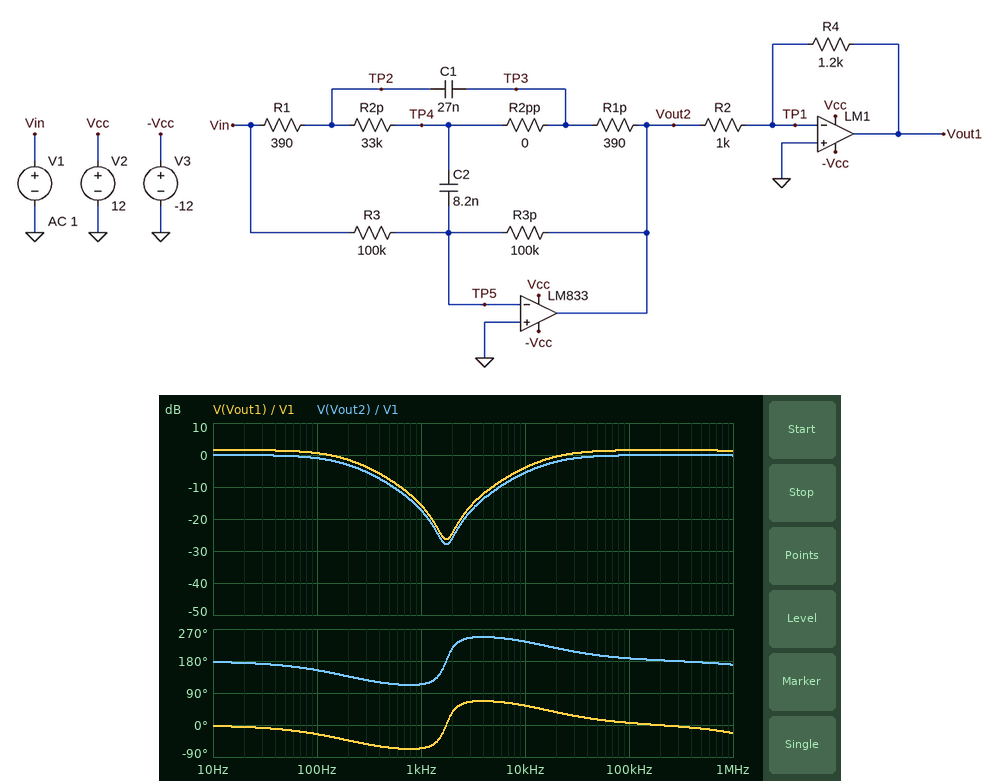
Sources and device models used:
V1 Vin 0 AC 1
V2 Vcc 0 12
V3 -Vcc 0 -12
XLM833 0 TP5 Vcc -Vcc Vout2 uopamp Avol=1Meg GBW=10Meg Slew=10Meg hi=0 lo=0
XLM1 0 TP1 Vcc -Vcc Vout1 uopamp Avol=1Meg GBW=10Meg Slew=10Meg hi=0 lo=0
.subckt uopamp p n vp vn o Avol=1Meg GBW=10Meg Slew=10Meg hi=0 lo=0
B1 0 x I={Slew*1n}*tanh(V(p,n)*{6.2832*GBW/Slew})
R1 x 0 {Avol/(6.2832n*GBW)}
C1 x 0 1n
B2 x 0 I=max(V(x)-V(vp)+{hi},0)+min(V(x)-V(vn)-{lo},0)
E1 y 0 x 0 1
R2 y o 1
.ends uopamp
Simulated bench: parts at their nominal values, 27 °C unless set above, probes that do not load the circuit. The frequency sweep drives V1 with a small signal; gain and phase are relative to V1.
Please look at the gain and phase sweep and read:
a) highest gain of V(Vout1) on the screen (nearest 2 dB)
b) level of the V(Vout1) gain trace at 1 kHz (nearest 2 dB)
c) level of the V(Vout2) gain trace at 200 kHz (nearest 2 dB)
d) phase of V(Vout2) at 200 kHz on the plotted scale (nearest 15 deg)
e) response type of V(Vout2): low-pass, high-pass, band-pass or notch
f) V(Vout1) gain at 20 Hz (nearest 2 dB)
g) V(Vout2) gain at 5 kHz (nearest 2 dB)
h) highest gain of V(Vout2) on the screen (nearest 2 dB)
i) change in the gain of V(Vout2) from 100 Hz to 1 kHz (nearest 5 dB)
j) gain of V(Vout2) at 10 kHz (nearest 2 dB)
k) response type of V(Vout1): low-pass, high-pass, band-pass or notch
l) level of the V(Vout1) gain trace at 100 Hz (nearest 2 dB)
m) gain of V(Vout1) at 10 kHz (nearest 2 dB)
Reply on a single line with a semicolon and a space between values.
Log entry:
2 dB; -16 dB; 0 dB; 180 deg; notch; 2 dB; -12 dB; 0 dB; -15 dB; -6 dB; notch; 0 dB; -4 dB
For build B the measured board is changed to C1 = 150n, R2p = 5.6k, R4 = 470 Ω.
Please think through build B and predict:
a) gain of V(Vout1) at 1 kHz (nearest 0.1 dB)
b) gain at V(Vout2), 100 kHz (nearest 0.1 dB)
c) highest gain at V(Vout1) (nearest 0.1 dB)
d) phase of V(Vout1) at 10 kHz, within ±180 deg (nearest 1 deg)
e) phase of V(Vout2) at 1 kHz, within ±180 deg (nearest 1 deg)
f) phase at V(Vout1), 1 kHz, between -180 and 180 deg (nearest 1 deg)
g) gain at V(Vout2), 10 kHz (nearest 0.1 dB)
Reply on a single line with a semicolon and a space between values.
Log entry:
-20.0 dB; 0 dB; -6.6 dB; 15 deg; -154 deg; 26 deg; -0.4 dB
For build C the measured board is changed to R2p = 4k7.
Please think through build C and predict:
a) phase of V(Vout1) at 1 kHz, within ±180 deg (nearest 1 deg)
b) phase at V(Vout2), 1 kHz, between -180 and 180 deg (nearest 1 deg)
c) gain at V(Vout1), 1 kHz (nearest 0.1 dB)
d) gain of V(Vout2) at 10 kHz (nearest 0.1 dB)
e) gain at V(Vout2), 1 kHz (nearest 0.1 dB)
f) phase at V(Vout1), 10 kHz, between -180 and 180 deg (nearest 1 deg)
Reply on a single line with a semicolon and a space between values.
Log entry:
-48 deg; 132 deg; -13.1 dB; -5.9 dB; -14.7 dB; 50 deg
